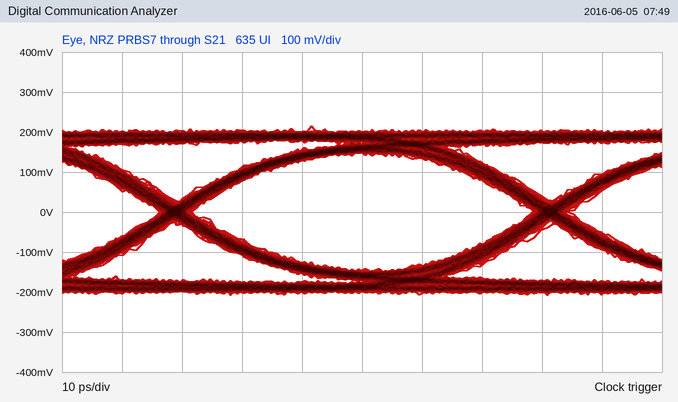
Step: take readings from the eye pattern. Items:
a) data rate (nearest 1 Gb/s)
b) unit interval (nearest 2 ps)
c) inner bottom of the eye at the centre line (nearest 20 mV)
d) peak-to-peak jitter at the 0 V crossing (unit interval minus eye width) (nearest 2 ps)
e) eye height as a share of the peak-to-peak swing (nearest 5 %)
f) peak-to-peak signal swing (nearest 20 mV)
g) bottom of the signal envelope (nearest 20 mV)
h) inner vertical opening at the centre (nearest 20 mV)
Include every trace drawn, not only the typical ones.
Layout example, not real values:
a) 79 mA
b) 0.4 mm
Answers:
a) 16 Gb/s
b) 62 ps
c) -140 mV
d) 6 ps
e) 70 %
f) 420 mV
g) -200 mV
h) 300 mV
